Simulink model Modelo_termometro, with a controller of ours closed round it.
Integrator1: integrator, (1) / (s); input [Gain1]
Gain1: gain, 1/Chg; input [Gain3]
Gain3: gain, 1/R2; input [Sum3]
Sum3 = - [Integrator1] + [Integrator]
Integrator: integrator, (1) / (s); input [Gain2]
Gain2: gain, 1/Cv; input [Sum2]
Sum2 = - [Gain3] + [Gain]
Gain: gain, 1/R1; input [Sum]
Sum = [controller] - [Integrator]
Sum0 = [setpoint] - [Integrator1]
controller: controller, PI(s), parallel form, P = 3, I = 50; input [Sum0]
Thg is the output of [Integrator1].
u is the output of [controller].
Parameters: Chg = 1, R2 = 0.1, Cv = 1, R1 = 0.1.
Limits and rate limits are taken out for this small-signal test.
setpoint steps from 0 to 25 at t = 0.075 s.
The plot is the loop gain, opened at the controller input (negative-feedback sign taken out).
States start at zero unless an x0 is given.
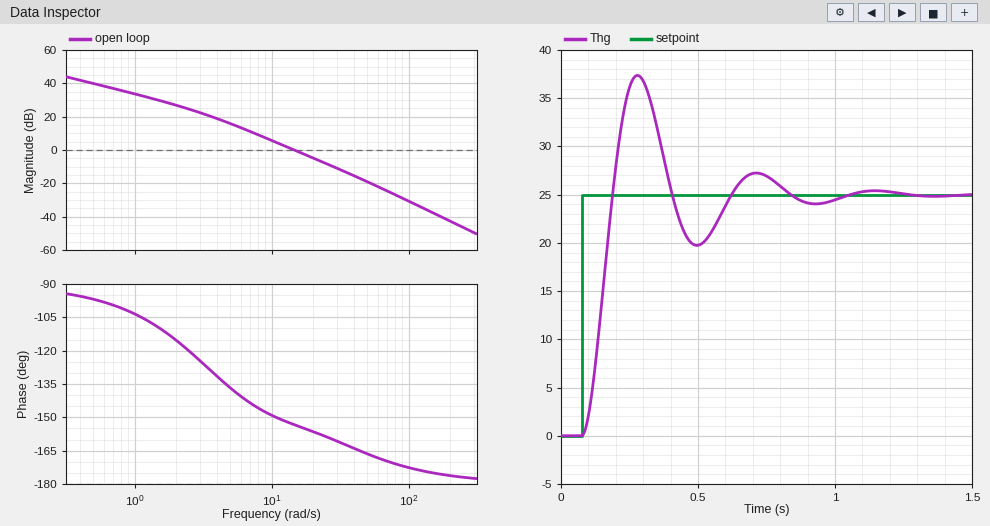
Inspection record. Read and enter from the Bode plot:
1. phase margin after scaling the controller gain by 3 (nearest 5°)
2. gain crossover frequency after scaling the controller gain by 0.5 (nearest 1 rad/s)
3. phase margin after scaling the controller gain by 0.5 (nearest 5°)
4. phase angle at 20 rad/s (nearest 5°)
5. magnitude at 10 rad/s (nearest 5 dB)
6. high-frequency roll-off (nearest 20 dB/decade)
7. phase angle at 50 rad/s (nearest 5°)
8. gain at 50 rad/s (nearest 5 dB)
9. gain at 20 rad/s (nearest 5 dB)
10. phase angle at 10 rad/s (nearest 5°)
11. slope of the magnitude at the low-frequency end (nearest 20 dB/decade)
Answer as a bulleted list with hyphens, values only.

- 20°
- 10 rad/s
- 30°
- -155°
- 5 dB
- -40 dB/decade
- -165°
- -20 dB
- -5 dB
- -150°
- -20 dB/decade
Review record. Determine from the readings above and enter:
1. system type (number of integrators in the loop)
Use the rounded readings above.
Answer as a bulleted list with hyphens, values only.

- 1
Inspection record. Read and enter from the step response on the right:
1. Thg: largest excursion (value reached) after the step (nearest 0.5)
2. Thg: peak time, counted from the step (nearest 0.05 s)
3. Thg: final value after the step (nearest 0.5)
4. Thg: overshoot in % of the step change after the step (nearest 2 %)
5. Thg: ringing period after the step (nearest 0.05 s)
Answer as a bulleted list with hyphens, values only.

- 37.5
- 0.20 s
- 25.0
- 50 %
- 0.45 s
